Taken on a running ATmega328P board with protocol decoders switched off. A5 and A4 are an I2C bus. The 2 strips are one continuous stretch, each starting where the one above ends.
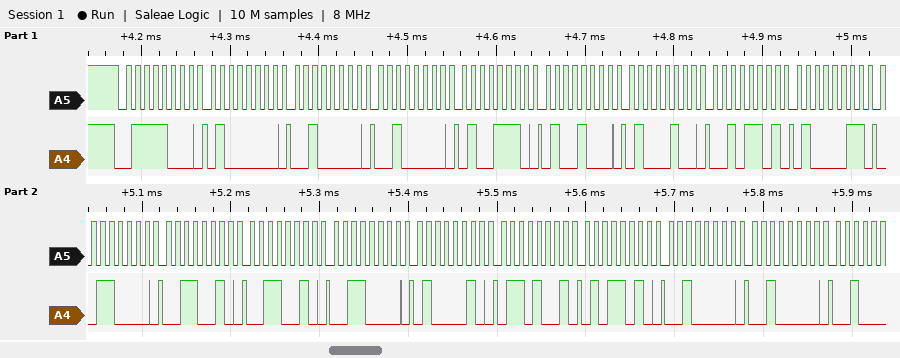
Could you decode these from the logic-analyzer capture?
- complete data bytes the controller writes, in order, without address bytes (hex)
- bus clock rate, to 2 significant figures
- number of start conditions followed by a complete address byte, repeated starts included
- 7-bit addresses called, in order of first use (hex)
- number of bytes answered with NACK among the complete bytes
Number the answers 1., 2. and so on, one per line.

1. 40 20 20 4E 48 44 2D 43 30 32 32 30 42 69 5A 20 20
2. 100 kHz
3. 1
4. 0x3C
5. 0
